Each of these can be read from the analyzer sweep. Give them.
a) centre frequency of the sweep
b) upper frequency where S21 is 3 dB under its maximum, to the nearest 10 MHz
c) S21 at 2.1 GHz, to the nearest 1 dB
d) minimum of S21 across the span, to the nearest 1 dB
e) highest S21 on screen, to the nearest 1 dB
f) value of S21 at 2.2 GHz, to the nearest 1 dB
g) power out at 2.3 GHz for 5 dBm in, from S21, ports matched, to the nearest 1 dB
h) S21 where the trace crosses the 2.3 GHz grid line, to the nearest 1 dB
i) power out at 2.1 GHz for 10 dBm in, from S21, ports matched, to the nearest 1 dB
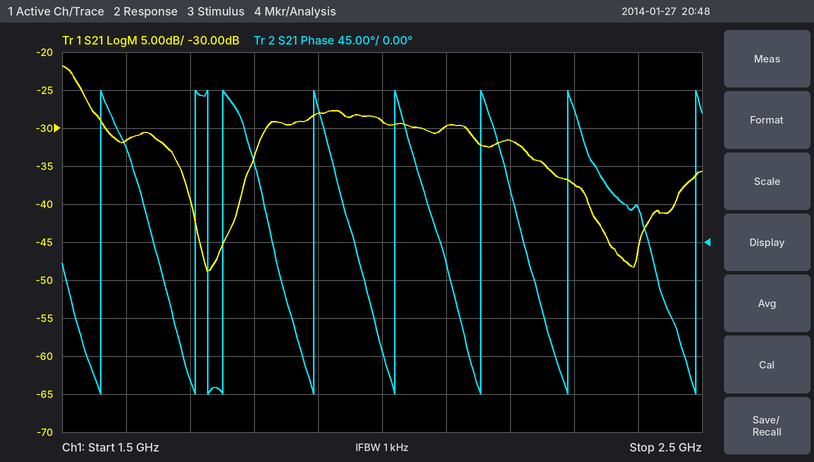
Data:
2 GHz
1.53 GHz
-30 dB
-49 dB
-22 dB
-32 dB
-32 dBm
-37 dB
-20 dBm
